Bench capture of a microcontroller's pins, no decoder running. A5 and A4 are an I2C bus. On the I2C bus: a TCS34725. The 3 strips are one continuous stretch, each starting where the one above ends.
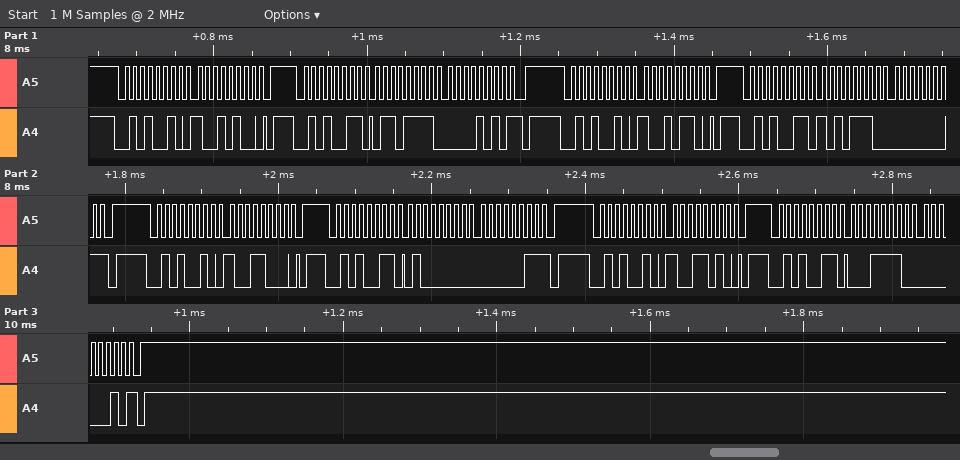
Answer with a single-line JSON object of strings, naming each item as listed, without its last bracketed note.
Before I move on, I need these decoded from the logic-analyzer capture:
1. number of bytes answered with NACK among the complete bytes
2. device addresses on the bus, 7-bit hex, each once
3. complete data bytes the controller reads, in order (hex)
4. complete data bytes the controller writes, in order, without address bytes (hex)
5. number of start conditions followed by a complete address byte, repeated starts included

{"number of bytes answered with NACK among the complete bytes": "4", "device addresses on the bus, 7-bit hex, each once": "0x29", "complete data bytes the controller reads, in order": "6F 0A AE 01 40 03 1E 02", "complete data bytes the controller writes, in order, without address bytes": "94 96 98 9A", "number of start conditions followed by a complete address byte, repeated starts included": "8"}
